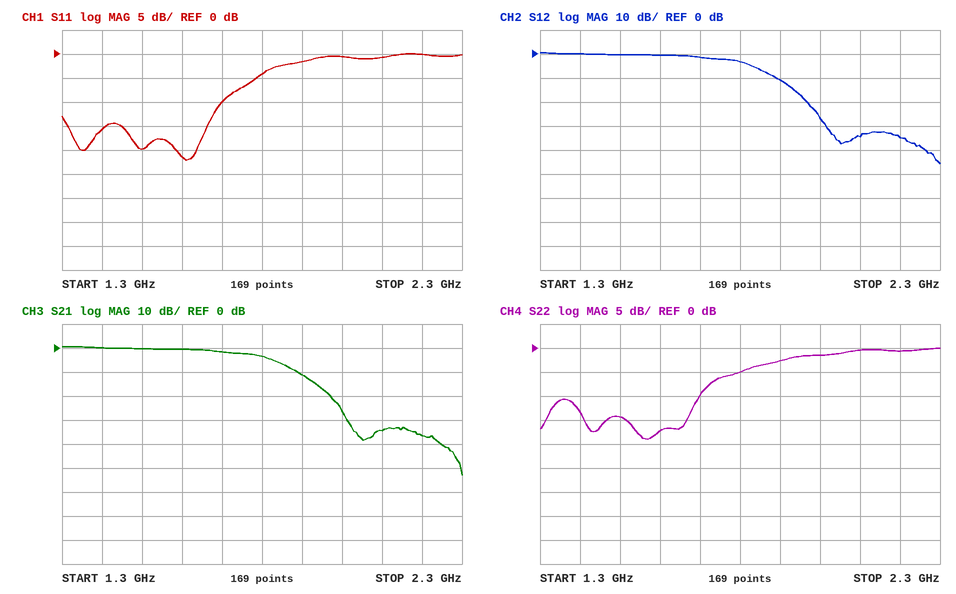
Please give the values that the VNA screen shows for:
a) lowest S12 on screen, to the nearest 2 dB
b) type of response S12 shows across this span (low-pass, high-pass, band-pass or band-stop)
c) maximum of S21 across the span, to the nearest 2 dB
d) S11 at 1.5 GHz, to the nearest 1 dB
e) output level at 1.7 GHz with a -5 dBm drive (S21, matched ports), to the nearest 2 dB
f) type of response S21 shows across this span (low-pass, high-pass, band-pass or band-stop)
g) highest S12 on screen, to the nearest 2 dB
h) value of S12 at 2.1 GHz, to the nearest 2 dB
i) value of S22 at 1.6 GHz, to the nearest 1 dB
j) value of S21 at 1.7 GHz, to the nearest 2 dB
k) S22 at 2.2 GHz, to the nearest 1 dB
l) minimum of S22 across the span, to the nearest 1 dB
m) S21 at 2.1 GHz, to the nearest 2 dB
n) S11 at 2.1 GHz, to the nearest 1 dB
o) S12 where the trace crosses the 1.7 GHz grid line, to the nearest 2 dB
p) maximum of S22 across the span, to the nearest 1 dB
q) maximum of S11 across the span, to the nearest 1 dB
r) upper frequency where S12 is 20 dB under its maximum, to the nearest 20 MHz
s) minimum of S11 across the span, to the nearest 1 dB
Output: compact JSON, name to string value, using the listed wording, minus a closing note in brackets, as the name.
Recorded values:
{"lowest S12 on screen, to the nearest 2 dB": "-46 dB", "type of response S12 shows across this span": "low-pass", "maximum of S21 across the span, to the nearest 2 dB": "0 dB", "S11 at 1.5 GHz, to the nearest 1 dB": "-20 dB", "output level at 1.7 GHz with a -5 dBm drive (S21, matched ports), to the nearest 2 dB": "-6 dBm", "type of response S21 shows across this span": "low-pass", "highest S12 on screen, to the nearest 2 dB": "0 dB", "value of S12 at 2.1 GHz, to the nearest 2 dB": "-34 dB", "value of S22 at 1.6 GHz, to the nearest 1 dB": "-17 dB", "value of S21 at 1.7 GHz, to the nearest 2 dB": "-2 dB", "S22 at 2.2 GHz, to the nearest 1 dB": "-1 dB", "minimum of S22 across the span, to the nearest 1 dB": "-19 dB", "S21 at 2.1 GHz, to the nearest 2 dB": "-34 dB", "S11 at 2.1 GHz, to the nearest 1 dB": "-1 dB", "S12 where the trace crosses the 1.7 GHz grid line, to the nearest 2 dB": "-2 dB", "maximum of S22 across the span, to the nearest 1 dB": "0 dB", "maximum of S11 across the span, to the nearest 1 dB": "0 dB", "upper frequency where S12 is 20 dB under its maximum, to the nearest 20 MHz": "1.96 GHz", "minimum of S11 across the span, to the nearest 1 dB": "-22 dB"}
